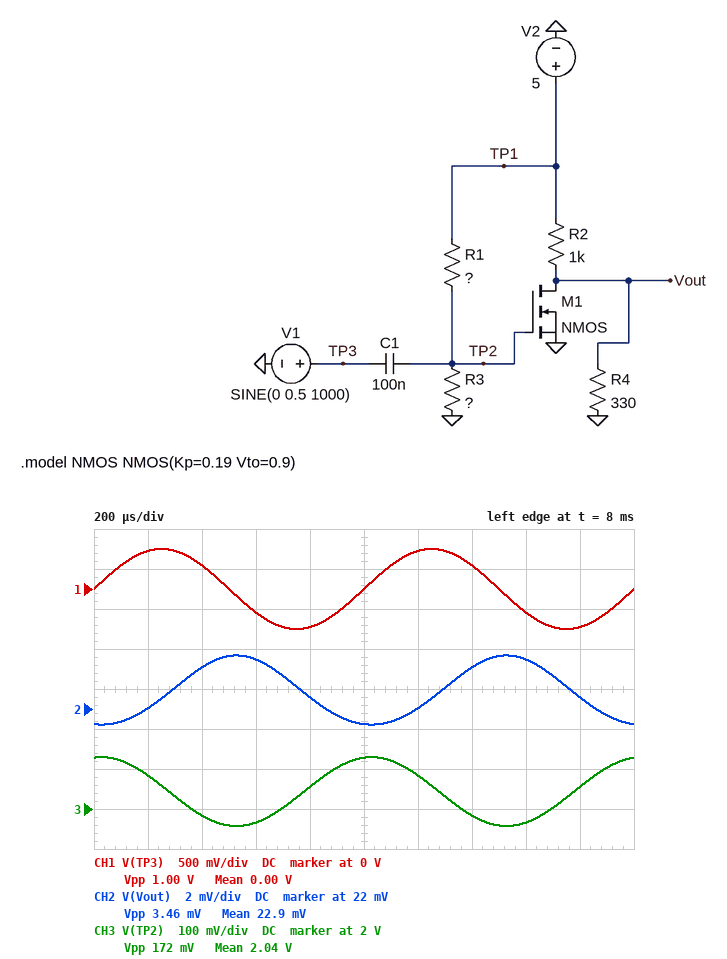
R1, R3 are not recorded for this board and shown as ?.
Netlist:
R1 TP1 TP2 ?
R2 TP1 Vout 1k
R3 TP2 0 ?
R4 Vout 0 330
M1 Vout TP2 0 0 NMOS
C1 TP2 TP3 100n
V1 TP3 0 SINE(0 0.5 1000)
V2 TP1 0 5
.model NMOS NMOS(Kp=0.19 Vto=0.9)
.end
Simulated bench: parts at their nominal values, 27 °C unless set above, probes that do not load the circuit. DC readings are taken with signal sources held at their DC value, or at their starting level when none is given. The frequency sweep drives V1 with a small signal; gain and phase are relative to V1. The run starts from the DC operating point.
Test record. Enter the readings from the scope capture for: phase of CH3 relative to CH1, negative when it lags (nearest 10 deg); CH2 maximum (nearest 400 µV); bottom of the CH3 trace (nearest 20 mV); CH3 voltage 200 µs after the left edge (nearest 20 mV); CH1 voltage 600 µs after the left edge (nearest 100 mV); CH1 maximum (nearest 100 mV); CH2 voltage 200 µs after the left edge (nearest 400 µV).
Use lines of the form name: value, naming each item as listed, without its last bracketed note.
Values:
phase of CH3 relative to CH1, negative when it lags: 80 deg
CH2 maximum: 24.8 mV
bottom of the CH3 trace: 1.96 V
CH3 voltage 200 µs after the left edge: 2.08 V
CH1 voltage 600 µs after the left edge: -300 mV
CH1 maximum: 500 mV
CH2 voltage 200 µs after the left edge: 22.0 mV
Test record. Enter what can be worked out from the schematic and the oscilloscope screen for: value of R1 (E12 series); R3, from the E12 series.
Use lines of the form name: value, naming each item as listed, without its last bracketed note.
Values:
value of R1: 680 Ω
R3, from the E12 series: 470 Ω
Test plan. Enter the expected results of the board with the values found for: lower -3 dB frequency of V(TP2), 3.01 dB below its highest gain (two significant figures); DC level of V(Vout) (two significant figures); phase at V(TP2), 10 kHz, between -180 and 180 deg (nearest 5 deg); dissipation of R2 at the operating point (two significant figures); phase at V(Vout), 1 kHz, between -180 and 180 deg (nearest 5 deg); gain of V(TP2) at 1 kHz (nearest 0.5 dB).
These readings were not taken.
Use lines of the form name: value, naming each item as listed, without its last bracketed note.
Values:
lower -3 dB frequency of V(TP2), 3.01 dB below its highest gain: 5.7 kHz
DC level of V(Vout): 23 mV
phase at V(TP2), 10 kHz, between -180 and 180 deg: 30 deg
dissipation of R2 at the operating point: 25 mW
phase at V(Vout), 1 kHz, between -180 and 180 deg: -100 deg
gain of V(TP2) at 1 kHz: -15.5 dB
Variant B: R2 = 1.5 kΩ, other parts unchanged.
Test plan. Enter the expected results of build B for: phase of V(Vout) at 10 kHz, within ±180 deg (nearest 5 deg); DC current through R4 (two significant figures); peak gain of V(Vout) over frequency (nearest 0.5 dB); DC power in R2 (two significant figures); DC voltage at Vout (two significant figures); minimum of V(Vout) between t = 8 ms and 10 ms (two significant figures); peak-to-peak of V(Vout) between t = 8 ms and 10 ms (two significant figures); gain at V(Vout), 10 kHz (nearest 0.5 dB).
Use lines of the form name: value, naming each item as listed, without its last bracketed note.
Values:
phase of V(Vout) at 10 kHz, within ±180 deg: -150 deg
DC current through R4: 46 µA
peak gain of V(Vout) over frequency: -37.5 dB
DC power in R2: 17 mW
DC voltage at Vout: 15 mV
minimum of V(Vout) between t = 8 ms and 10 ms: 14 mV
peak-to-peak of V(Vout) between t = 8 ms and 10 ms: 2.3 mV
gain at V(Vout), 10 kHz: -39.0 dB
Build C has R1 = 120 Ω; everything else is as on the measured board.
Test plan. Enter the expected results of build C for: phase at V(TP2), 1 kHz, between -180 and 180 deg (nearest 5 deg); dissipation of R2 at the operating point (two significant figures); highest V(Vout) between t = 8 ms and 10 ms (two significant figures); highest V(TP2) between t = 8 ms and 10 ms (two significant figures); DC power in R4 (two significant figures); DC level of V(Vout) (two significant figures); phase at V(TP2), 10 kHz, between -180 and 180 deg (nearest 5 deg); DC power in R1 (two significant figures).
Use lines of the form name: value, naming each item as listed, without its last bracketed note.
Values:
phase at V(TP2), 1 kHz, between -180 and 180 deg: 85 deg
dissipation of R2 at the operating point: 25 mW
highest V(Vout) between t = 8 ms and 10 ms: 8.6 mV
highest V(TP2) between t = 8 ms and 10 ms: 4.0 V
DC power in R4: 220 nW
DC level of V(Vout): 8.5 mV
phase at V(TP2), 10 kHz, between -180 and 180 deg: 60 deg
DC power in R1: 8.6 mW
